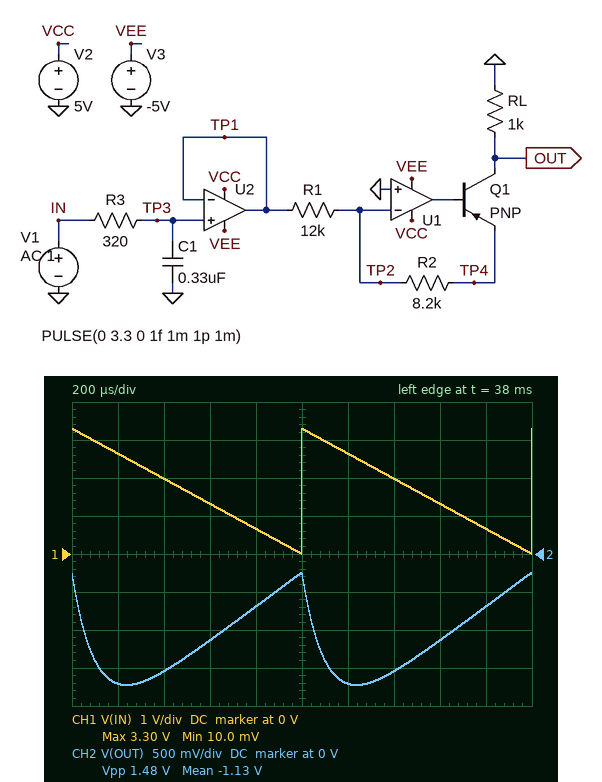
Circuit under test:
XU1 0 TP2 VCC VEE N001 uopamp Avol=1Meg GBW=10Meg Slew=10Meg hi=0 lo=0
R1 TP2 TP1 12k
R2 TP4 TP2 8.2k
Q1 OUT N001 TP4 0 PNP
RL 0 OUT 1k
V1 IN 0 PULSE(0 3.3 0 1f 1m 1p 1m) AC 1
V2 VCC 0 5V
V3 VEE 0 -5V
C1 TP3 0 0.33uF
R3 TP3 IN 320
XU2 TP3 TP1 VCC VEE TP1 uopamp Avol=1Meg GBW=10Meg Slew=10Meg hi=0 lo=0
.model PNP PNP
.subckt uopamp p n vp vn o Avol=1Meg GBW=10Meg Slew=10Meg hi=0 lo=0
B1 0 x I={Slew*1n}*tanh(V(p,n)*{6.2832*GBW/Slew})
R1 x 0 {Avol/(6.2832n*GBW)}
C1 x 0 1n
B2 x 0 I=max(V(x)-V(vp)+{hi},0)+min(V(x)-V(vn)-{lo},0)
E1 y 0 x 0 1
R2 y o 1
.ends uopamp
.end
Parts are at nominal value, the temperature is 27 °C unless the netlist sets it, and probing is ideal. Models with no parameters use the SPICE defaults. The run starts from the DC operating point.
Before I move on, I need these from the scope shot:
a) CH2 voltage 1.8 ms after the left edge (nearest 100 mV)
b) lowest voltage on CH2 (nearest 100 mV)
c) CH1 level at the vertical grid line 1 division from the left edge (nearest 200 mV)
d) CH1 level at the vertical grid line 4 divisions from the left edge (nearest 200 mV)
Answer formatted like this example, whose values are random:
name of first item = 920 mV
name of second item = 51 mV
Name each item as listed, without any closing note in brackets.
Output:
CH2 voltage 1.8 ms after the left edge = -700 mV
lowest voltage on CH2 = -1.7 V
CH1 level at the vertical grid line 1 division from the left edge = 2.6 V
CH1 level at the vertical grid line 4 divisions from the left edge = 600 mV
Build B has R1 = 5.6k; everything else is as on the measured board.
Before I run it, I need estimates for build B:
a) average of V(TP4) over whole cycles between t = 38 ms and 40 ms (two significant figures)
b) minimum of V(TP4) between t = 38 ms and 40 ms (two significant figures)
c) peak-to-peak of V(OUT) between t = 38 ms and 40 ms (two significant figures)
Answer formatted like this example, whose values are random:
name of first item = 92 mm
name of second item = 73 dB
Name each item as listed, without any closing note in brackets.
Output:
average of V(TP4) over whole cycles between t = 38 ms and 40 ms = -2.4 V
minimum of V(TP4) between t = 38 ms and 40 ms = -3.7 V
peak-to-peak of V(OUT) between t = 38 ms and 40 ms = 3.2 V
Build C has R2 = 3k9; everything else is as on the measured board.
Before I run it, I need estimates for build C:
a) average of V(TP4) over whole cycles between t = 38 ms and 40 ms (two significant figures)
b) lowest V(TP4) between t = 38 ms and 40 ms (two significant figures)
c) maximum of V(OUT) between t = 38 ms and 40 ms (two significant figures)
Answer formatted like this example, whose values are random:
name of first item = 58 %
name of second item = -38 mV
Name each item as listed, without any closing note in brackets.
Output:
average of V(TP4) over whole cycles between t = 38 ms and 40 ms = -540 mV
lowest V(TP4) between t = 38 ms and 40 ms = -820 mV
maximum of V(OUT) between t = 38 ms and 40 ms = -120 mV
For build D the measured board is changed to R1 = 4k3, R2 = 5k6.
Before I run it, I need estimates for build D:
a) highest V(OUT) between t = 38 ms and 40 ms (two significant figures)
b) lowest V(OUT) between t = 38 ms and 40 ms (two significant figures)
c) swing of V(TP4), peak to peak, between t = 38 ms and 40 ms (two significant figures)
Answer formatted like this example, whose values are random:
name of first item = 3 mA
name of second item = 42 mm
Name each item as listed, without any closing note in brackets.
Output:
highest V(OUT) between t = 38 ms and 40 ms = -460 mV
lowest V(OUT) between t = 38 ms and 40 ms = -3.3 V
swing of V(TP4), peak to peak, between t = 38 ms and 40 ms = 2.8 V
